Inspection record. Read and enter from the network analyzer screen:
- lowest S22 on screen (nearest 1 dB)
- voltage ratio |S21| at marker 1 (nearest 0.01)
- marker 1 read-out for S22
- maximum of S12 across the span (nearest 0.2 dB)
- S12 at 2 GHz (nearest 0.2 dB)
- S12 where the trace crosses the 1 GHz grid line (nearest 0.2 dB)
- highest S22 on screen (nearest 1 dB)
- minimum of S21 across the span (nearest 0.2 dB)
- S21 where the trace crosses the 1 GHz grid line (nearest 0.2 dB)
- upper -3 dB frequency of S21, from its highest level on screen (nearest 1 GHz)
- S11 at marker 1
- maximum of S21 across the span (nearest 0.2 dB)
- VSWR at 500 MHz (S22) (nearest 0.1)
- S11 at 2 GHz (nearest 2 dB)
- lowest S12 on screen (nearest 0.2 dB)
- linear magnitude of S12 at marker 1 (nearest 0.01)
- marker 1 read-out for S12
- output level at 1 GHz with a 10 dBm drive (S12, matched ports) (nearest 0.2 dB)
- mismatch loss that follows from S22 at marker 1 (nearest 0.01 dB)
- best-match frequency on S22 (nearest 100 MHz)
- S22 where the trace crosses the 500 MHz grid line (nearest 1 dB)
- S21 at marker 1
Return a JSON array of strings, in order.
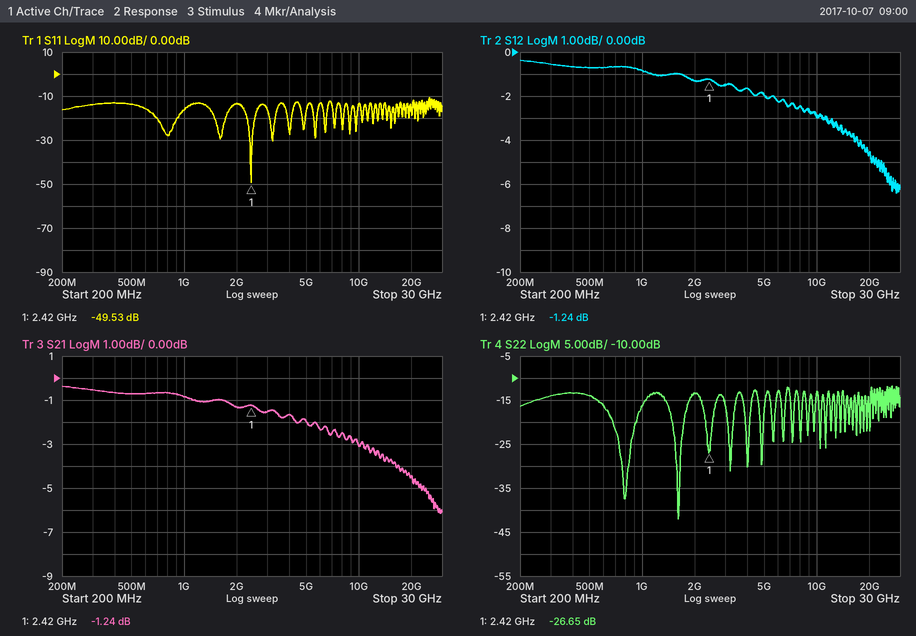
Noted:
["-42 dB", "0.87", "-26.65 dB", "-0.4 dB", "-1.4 dB", "-0.8 dB", "-12 dB", "-6.2 dB", "-0.8 dB", "12 GHz", "-49.53 dB", "-0.4 dB", "1.5", "-14 dB", "-6.4 dB", "0.87", "-1.24 dB", "9.2 dBm", "0.01 dB", "1.6 GHz", "-14 dB", "-1.24 dB"]
